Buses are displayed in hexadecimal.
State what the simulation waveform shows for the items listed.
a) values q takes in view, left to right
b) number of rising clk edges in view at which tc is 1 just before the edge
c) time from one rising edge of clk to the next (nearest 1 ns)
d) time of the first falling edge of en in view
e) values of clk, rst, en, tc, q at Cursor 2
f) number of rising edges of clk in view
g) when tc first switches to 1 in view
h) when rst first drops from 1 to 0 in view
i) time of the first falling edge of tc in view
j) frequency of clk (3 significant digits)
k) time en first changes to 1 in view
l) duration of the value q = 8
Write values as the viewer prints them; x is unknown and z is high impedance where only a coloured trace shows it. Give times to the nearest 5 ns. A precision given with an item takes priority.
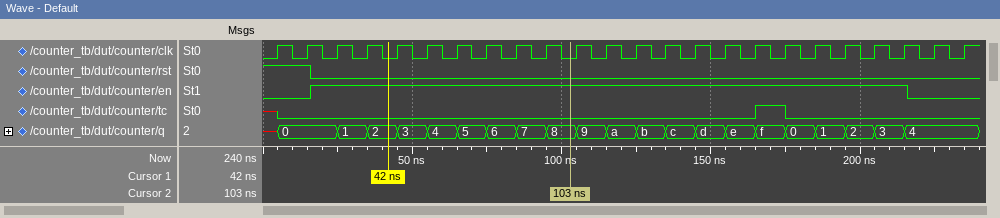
x, 0, 1, 2, 3, 4, 5, 6, 7, 8, 9, a, b, c, d, e, f, 0, 1, 2, 3, 4
1
10 ns
215 ns
clk=0, rst=0, en=1, tc=0, q=8
24
165 ns
15 ns
175 ns
100 MHz
15 ns
10 ns
